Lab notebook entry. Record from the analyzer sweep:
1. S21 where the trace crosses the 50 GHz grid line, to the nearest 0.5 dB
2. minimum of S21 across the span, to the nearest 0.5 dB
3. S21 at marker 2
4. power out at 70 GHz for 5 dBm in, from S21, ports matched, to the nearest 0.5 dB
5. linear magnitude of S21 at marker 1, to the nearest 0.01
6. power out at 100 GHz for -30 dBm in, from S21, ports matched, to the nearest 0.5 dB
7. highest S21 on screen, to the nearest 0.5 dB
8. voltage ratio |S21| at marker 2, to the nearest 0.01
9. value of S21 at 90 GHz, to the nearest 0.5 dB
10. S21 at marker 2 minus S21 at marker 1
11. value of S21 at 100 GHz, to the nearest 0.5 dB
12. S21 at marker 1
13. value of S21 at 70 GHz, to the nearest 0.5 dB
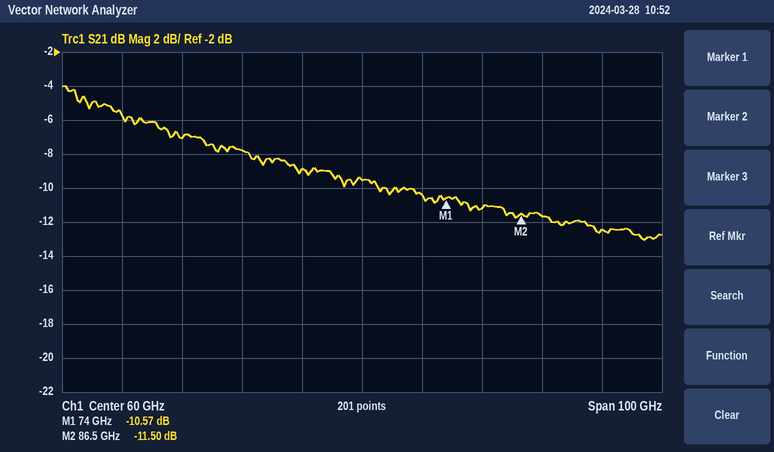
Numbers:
-9.0 dB
-13.0 dB
-11.50 dB
-5.5 dBm
0.30
-42.5 dBm
-4.0 dB
0.27
-11.5 dB
-0.93 dB
-12.5 dB
-10.57 dB
-10.5 dB
